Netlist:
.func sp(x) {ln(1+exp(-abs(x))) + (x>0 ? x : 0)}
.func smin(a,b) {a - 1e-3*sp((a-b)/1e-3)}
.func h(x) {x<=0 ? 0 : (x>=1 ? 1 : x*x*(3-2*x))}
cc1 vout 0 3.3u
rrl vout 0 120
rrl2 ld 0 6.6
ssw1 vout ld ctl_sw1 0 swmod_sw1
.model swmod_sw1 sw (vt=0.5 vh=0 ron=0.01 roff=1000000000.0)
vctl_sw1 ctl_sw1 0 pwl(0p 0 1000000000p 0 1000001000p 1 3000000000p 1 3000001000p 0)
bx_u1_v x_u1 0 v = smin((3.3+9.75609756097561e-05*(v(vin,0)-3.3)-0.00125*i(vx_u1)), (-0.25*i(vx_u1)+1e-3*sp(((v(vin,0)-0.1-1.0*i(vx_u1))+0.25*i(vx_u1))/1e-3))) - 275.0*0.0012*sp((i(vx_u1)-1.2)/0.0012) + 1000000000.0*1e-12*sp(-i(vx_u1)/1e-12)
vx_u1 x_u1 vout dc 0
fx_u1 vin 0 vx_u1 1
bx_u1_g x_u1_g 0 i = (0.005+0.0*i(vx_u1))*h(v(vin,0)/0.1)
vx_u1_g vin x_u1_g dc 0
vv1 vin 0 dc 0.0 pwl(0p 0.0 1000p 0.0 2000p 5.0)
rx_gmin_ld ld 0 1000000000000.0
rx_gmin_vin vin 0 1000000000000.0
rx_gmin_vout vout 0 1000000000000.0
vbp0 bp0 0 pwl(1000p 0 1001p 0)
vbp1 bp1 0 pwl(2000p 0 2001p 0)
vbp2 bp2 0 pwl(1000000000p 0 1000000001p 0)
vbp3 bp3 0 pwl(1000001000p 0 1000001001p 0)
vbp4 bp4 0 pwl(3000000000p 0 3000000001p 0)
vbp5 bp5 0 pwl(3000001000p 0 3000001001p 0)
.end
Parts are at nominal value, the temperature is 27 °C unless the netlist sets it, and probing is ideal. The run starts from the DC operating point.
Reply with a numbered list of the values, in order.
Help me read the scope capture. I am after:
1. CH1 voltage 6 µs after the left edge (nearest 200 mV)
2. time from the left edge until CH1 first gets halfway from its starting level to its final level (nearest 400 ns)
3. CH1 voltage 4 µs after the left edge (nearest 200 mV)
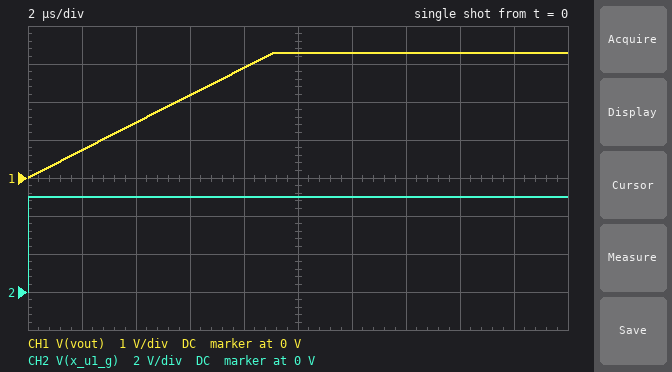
1. 2.2 V
2. 4.4 µs
3. 1.4 V
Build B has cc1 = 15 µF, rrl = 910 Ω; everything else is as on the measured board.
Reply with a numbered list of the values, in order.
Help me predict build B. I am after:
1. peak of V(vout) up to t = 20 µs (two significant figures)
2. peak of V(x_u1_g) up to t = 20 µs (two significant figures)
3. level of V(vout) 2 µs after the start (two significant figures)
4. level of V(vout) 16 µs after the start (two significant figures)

1. 1.6 V
2. 5.0 V
3. 160 mV
4. 1.3 V
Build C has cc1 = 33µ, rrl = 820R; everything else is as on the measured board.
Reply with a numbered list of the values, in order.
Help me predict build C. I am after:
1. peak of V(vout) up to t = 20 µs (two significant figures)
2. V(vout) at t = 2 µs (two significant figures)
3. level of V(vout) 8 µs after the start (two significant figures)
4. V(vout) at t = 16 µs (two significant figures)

1. 730 mV
2. 73 mV
3. 290 mV
4. 590 mV
